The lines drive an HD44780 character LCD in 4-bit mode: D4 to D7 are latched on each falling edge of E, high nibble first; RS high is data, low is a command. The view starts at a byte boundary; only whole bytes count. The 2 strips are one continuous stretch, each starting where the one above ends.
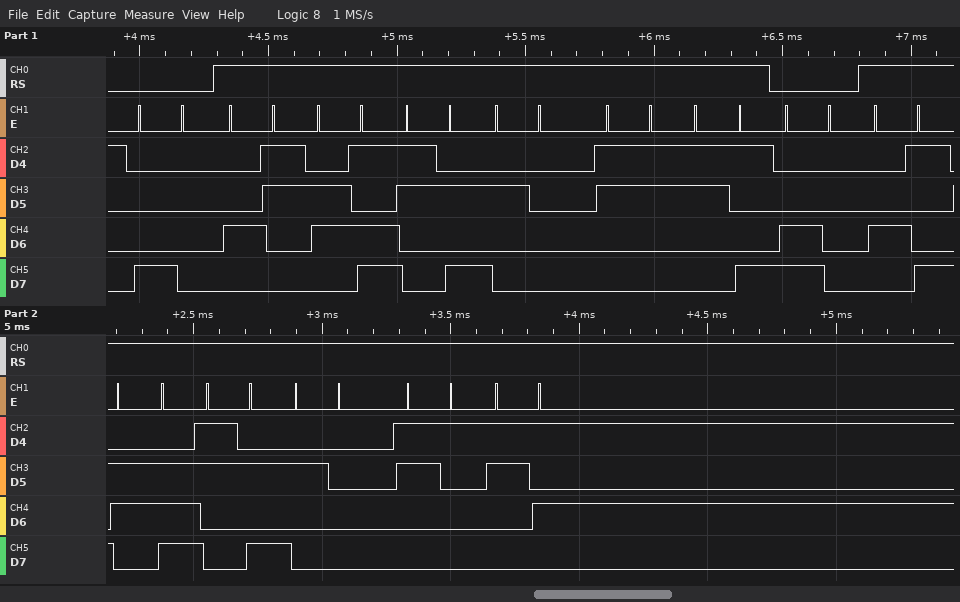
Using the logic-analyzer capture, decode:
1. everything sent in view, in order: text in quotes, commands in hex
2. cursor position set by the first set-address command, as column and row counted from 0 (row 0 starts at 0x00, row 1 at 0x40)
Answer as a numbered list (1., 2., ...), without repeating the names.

1. 0x80 "Cm: 39" 0xC0 "In: 15"
2. column 0, row 0
